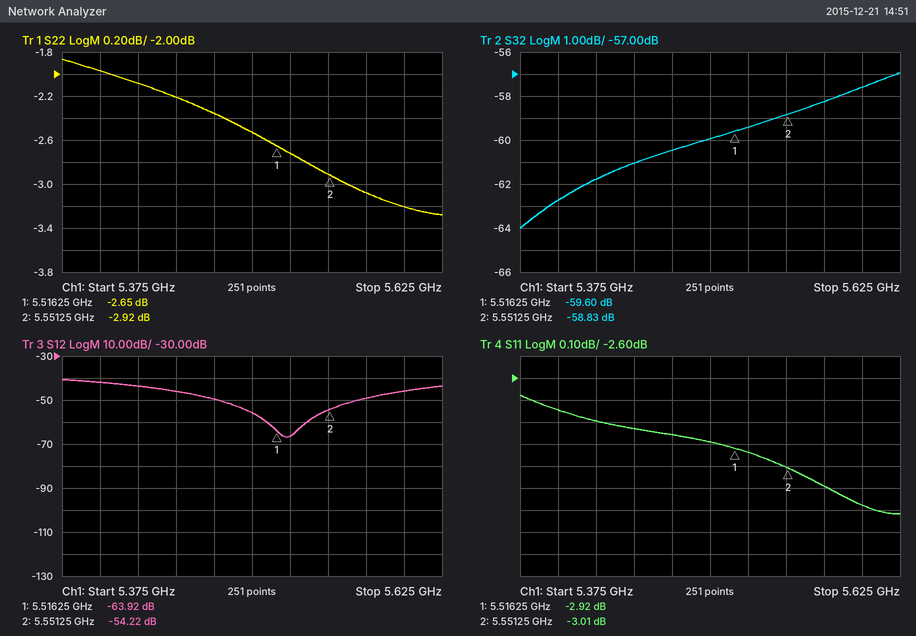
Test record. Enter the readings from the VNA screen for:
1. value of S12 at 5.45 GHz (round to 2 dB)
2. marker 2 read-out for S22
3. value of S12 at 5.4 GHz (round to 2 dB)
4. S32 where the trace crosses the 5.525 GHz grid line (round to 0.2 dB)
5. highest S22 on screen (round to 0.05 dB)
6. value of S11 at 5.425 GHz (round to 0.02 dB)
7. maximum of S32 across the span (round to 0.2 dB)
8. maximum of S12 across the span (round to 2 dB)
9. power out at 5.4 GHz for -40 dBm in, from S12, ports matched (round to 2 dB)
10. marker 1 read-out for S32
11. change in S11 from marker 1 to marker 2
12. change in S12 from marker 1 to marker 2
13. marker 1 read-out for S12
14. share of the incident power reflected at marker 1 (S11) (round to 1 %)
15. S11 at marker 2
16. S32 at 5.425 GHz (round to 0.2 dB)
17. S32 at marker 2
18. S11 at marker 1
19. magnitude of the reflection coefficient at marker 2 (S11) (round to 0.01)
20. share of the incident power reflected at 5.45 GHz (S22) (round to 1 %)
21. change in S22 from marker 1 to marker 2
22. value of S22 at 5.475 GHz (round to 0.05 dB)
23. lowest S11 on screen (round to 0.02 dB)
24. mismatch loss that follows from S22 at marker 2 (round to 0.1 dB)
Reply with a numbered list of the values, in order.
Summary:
1. -46 dB
2. -2.92 dB
3. -42 dB
4. -59.4 dB
5. -1.85 dB
6. -2.80 dB
7. -57.0 dB
8. -40 dB
9. -82 dBm
10. -59.60 dB
11. -0.09 dB
12. 9.70 dB
13. -63.92 dB
14. 51 %
15. -3.01 dB
16. -61.8 dB
17. -58.83 dB
18. -2.92 dB
19. 0.71
20. 60 %
21. -0.27 dB
22. -2.35 dB
23. -3.22 dB
24. 3.1 dB
